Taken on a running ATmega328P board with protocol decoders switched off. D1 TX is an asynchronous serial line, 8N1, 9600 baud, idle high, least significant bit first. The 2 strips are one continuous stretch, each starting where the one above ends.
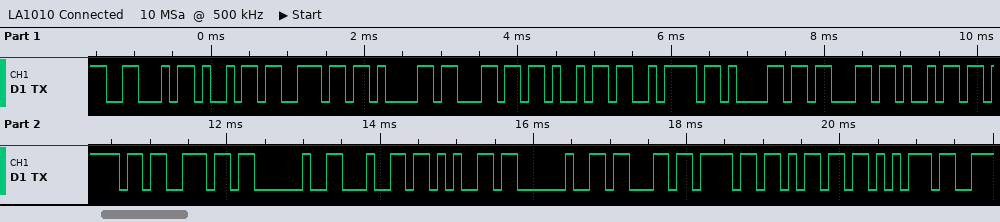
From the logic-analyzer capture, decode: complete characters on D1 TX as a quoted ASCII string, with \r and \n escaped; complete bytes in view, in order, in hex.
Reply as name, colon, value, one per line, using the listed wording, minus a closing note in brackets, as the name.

complete characters on D1 TX as a quoted ASCII string, with \r and \n escaped: "Finalizacion de comu"
complete bytes in view, in order, in hex: 46 69 6E 61 6C 69 7A 61 63 69 6F 6E 20 64 65 20 63 6F 6D 75
